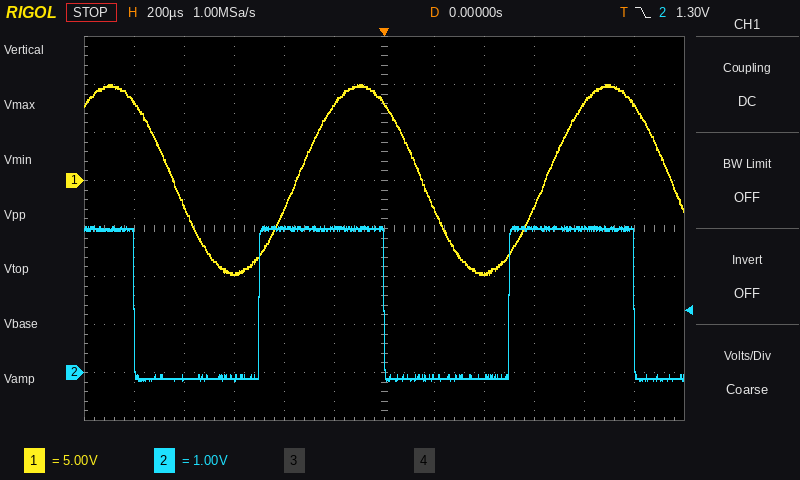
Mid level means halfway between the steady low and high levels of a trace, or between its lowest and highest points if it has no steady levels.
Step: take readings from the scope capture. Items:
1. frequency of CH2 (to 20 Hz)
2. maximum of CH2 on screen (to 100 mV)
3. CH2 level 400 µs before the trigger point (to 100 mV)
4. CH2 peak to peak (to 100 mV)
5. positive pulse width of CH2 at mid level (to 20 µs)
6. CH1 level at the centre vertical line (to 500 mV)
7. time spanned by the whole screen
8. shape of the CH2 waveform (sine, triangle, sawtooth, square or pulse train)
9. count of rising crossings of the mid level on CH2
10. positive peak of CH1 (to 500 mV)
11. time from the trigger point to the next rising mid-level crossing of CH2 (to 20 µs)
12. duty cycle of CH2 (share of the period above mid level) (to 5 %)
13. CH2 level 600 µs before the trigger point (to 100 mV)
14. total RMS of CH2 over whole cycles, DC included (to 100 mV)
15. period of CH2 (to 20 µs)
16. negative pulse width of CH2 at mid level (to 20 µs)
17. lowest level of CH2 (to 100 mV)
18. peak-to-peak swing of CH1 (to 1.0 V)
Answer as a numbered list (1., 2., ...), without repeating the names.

1. 1.00 kHz
2. 3.0 V
3. 3.0 V
4. 3.2 V
5. 500 µs
6. 8.0 V
7. 2.4 ms
8. square
9. 2
10. 10.0 V
11. 500 µs
12. 50 %
13. -100 mV
14. 2.1 V
15. 1.00 ms
16. 500 µs
17. -200 mV
18. 20.0 V
